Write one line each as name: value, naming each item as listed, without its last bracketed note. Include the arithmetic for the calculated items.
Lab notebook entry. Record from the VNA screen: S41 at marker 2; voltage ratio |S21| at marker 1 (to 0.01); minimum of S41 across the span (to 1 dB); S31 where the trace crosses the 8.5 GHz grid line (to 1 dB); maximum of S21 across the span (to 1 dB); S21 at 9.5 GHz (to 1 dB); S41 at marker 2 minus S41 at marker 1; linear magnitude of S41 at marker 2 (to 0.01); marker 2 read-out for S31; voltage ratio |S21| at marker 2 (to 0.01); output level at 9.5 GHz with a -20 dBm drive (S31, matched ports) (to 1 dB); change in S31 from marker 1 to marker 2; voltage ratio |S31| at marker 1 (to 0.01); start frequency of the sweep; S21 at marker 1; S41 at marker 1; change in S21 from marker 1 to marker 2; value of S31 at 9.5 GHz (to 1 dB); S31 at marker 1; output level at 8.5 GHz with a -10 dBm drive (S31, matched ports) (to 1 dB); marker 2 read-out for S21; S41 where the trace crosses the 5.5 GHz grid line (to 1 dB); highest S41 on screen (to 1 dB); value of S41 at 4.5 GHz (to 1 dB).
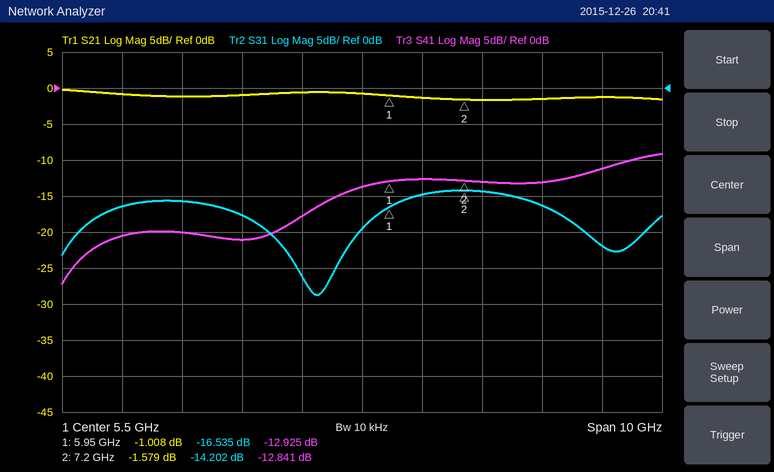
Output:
S41 at marker 2: -12.841 dB
voltage ratio |S21| at marker 1: 10^(-1.008/20) ≈ 0.89
minimum of S41 across the span: -27 dB
S31 where the trace crosses the 8.5 GHz grid line: -16 dB
maximum of S21 across the span: 0 dB
S21 at 9.5 GHz: -1 dB
S41 at marker 2 minus S41 at marker 1: -12.841 − (-12.925) = 0.084 dB
linear magnitude of S41 at marker 2: 10^(-12.841/20) ≈ 0.23
marker 2 read-out for S31: -14.202 dB
voltage ratio |S21| at marker 2: 10^(-1.579/20) ≈ 0.83
output level at 9.5 GHz with a -20 dBm drive (S31, matched ports): -20 dBm + (-22 dB) = -42 dBm
change in S31 from marker 1 to marker 2: -14.202 − (-16.535) = 2.333 dB
voltage ratio |S31| at marker 1: 10^(-16.535/20) ≈ 0.15
start frequency of the sweep: 500 MHz
S21 at marker 1: -1.008 dB
S41 at marker 1: -12.925 dB
change in S21 from marker 1 to marker 2: -1.579 − (-1.008) = -0.571 dB
value of S31 at 9.5 GHz: -22 dB
S31 at marker 1: -16.535 dB
output level at 8.5 GHz with a -10 dBm drive (S31, matched ports): -10 dBm + (-16 dB) = -26 dBm
marker 2 read-out for S21: -1.579 dB
S41 where the trace crosses the 5.5 GHz grid line: -14 dB
highest S41 on screen: -9 dB
value of S41 at 4.5 GHz: -18 dB
